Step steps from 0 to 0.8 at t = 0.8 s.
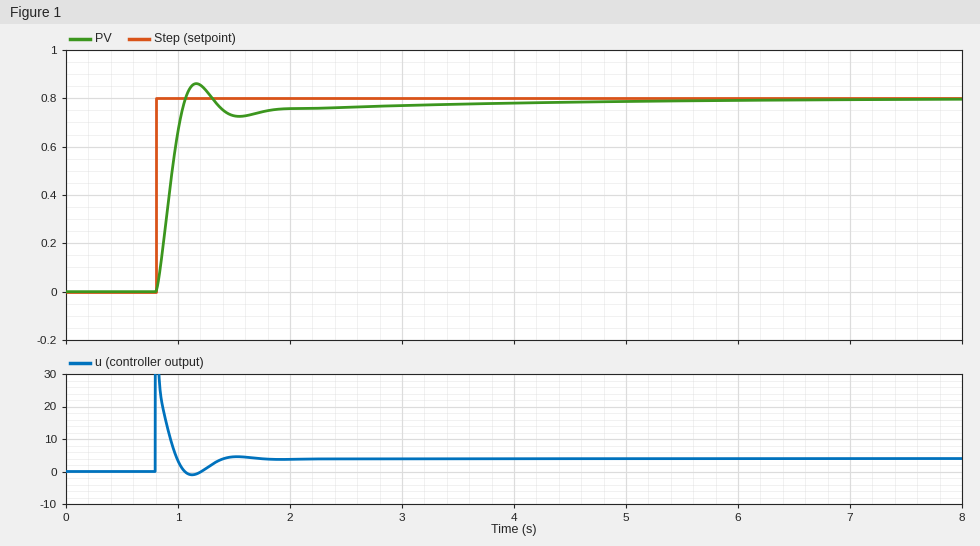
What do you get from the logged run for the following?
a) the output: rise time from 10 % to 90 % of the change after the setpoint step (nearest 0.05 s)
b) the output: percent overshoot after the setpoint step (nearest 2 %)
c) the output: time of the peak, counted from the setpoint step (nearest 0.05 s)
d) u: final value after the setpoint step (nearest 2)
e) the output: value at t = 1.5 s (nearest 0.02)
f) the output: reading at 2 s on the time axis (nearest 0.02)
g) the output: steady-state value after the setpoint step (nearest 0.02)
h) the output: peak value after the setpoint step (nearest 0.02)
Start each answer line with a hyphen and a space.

- 0.20 s
- 8 %
- 0.35 s
- 4
- 0.72
- 0.76
- 0.80
- 0.86
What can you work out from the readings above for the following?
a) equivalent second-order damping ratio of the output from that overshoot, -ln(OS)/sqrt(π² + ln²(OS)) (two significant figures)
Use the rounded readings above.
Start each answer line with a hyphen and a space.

- 0.63
